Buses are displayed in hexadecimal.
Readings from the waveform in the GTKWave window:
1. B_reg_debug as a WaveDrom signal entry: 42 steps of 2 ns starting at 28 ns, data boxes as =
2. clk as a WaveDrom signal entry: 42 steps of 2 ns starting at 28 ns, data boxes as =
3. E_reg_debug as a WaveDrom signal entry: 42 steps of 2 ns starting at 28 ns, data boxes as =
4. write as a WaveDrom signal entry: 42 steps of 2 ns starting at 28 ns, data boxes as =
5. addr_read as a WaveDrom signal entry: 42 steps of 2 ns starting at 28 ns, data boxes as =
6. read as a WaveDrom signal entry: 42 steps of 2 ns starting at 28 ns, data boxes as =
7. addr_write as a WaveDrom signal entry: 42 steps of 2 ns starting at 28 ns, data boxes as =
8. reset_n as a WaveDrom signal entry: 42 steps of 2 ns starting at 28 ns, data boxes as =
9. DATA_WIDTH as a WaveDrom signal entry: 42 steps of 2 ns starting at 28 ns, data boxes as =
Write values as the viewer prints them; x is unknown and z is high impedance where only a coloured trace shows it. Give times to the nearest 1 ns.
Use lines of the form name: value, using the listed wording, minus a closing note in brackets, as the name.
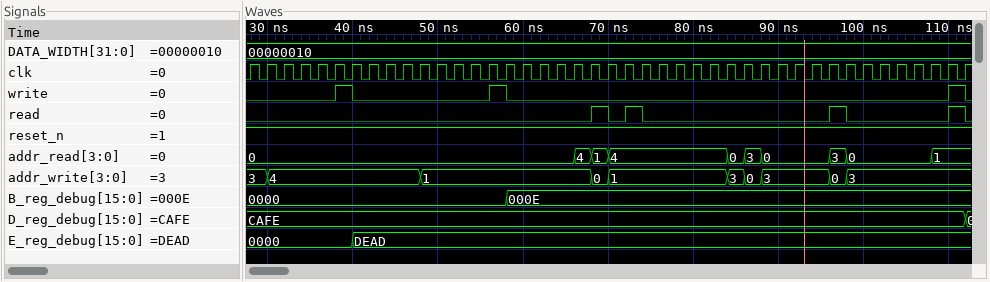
B_reg_debug as a WaveDrom signal entry: 42 steps of 2 ns starting at 28 ns, data boxes as =: {name: 'B_reg_debug', wave: '=..............=..........................', data: '0000 000E'}
clk as a WaveDrom signal entry: 42 steps of 2 ns starting at 28 ns, data boxes as =: {name: 'clk', wave: 'p.........................................'}
E_reg_debug as a WaveDrom signal entry: 42 steps of 2 ns starting at 28 ns, data boxes as =: {name: 'E_reg_debug', wave: '=.....=...................................', data: '0000 DEAD'}
write as a WaveDrom signal entry: 42 steps of 2 ns starting at 28 ns, data boxes as =: {name: 'write', wave: '0....10.......10.........................1'}
addr_read as a WaveDrom signal entry: 42 steps of 2 ns starting at 28 ns, data boxes as =: {name: 'addr_read', wave: '=..................===......===...==....=.', data: '0 4 1 4 0 3 0 3 0 1'}
read as a WaveDrom signal entry: 42 steps of 2 ns starting at 28 ns, data boxes as =: {name: 'read', wave: '0...................1010..........10.....1'}
addr_write as a WaveDrom signal entry: 42 steps of 2 ns starting at 28 ns, data boxes as =: {name: 'addr_write', wave: '==........=.........==......===...==......', data: '3 4 1 0 1 3 0 3 0 3'}
reset_n as a WaveDrom signal entry: 42 steps of 2 ns starting at 28 ns, data boxes as =: {name: 'reset_n', wave: '1.........................................'}
DATA_WIDTH as a WaveDrom signal entry: 42 steps of 2 ns starting at 28 ns, data boxes as =: {name: 'DATA_WIDTH', wave: '=.........................................', data: '00000010'}
